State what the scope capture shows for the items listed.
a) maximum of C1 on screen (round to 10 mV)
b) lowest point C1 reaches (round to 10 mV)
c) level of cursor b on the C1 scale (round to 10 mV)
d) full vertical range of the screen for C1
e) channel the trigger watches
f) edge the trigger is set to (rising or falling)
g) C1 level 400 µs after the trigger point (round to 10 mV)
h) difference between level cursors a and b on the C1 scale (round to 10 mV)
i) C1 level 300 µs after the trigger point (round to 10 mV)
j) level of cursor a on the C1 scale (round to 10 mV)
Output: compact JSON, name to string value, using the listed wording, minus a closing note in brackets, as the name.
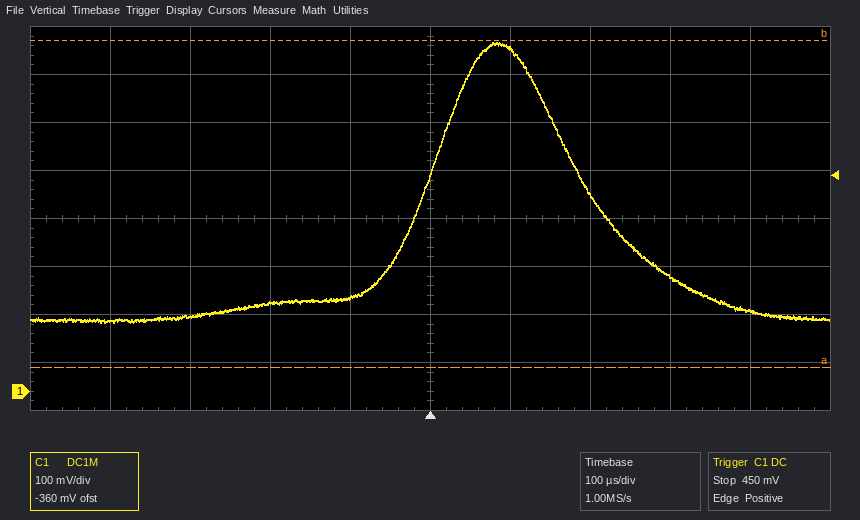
{"maximum of C1 on screen": "730 mV", "lowest point C1 reaches": "140 mV", "level of cursor b on the C1 scale": "730 mV", "full vertical range of the screen for C1": "800 mV", "channel the trigger watches": "C1", "edge the trigger is set to": "rising", "C1 level 400 µs after the trigger point": "170 mV", "difference between level cursors a and b on the C1 scale": "680 mV", "C1 level 300 µs after the trigger point": "240 mV", "level of cursor a on the C1 scale": "50 mV"}
